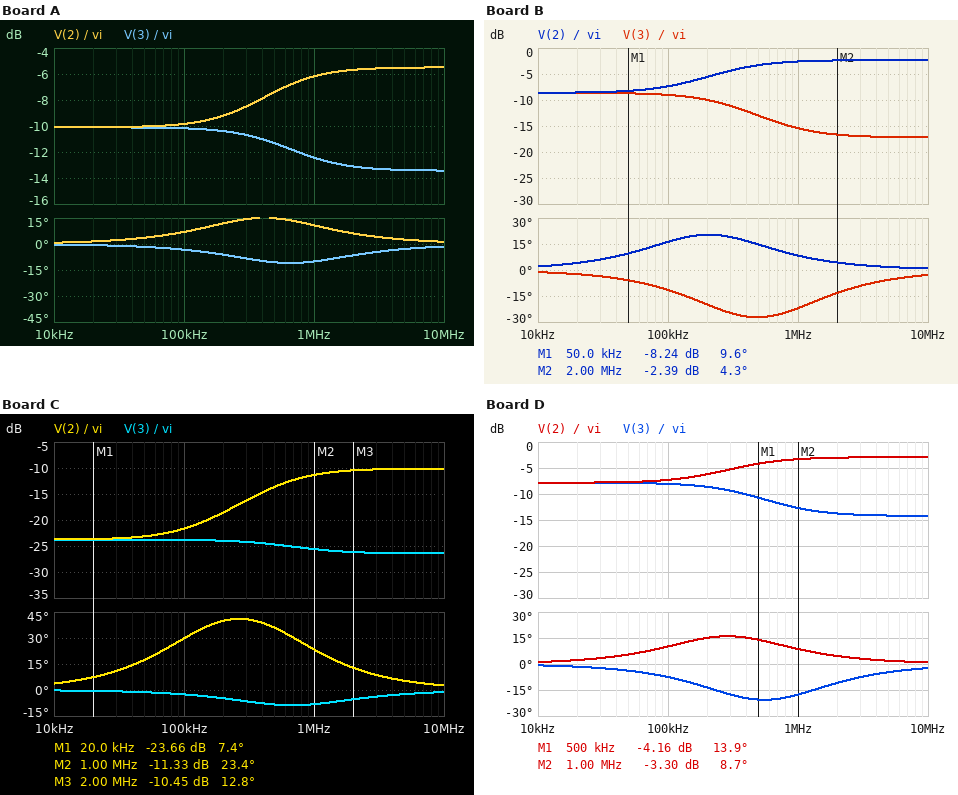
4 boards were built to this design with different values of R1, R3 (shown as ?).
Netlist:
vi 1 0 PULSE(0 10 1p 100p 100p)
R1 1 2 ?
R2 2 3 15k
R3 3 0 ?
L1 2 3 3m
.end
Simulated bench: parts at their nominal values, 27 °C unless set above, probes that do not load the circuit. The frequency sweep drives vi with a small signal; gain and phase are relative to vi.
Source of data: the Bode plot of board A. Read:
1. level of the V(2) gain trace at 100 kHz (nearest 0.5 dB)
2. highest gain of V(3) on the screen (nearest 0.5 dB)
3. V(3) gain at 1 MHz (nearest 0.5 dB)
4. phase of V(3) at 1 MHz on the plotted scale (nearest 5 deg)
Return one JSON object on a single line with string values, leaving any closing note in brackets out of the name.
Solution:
{"level of the V(2) gain trace at 100 kHz": "-10.0 dB", "highest gain of V(3) on the screen": "-10.0 dB", "V(3) gain at 1 MHz": "-12.5 dB", "phase of V(3) at 1 MHz on the plotted scale": "-10 deg"}
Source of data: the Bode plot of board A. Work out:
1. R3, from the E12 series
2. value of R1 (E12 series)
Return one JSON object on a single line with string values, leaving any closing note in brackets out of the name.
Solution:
{"R3, from the E12 series": "10 kΩ", "value of R1": "22 kΩ"}
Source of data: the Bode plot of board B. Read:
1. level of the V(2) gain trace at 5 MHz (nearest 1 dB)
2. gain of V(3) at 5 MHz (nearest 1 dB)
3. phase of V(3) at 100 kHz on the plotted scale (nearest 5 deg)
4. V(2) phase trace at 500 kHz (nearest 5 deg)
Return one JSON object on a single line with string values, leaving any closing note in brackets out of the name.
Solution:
{"level of the V(2) gain trace at 5 MHz": "-2 dB", "gain of V(3) at 5 MHz": "-17 dB", "phase of V(3) at 100 kHz on the plotted scale": "-10 deg", "V(2) phase trace at 500 kHz": "15 deg"}
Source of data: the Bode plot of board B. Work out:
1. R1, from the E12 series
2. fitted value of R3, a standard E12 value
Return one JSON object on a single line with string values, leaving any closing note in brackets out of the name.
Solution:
{"R1, from the E12 series": "5.6 kΩ", "fitted value of R3, a standard E12 value": "3.3 kΩ"}
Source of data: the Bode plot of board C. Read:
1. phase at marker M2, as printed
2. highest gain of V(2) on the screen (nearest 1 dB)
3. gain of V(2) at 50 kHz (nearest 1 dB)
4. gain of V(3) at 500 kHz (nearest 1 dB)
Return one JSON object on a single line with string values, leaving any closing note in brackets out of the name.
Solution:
{"phase at marker M2, as printed": "23.4 deg", "highest gain of V(2) on the screen": "-10 dB", "gain of V(2) at 50 kHz": "-23 dB", "gain of V(3) at 500 kHz": "-25 dB"}
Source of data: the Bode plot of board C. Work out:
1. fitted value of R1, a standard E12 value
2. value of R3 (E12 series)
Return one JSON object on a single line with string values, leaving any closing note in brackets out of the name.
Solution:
{"fitted value of R1, a standard E12 value": "39 kΩ", "value of R3": "2.7 kΩ"}
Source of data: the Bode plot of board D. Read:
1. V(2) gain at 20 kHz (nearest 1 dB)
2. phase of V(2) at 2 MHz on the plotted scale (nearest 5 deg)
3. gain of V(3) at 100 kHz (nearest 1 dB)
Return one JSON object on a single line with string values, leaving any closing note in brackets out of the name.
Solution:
{"V(2) gain at 20 kHz": "-8 dB", "phase of V(2) at 2 MHz on the plotted scale": "5 deg", "gain of V(3) at 100 kHz": "-8 dB"}
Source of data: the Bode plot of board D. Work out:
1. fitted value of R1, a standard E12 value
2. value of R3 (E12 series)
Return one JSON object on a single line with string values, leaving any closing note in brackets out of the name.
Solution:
{"fitted value of R1, a standard E12 value": "8.2 kΩ", "value of R3": "5.6 kΩ"}
